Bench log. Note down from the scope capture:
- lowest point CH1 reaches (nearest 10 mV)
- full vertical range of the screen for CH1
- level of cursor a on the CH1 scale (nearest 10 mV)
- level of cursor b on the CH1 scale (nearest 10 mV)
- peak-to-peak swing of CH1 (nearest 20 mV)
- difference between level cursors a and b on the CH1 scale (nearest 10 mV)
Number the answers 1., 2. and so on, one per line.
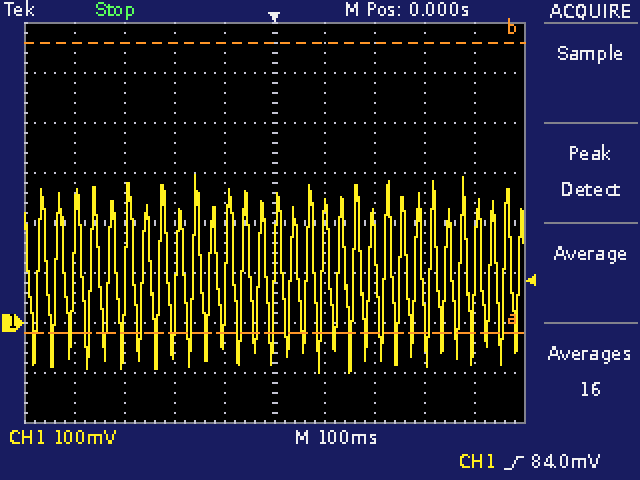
1. -100 mV
2. 800 mV
3. -20 mV
4. 560 mV
5. 400 mV
6. 580 mV
